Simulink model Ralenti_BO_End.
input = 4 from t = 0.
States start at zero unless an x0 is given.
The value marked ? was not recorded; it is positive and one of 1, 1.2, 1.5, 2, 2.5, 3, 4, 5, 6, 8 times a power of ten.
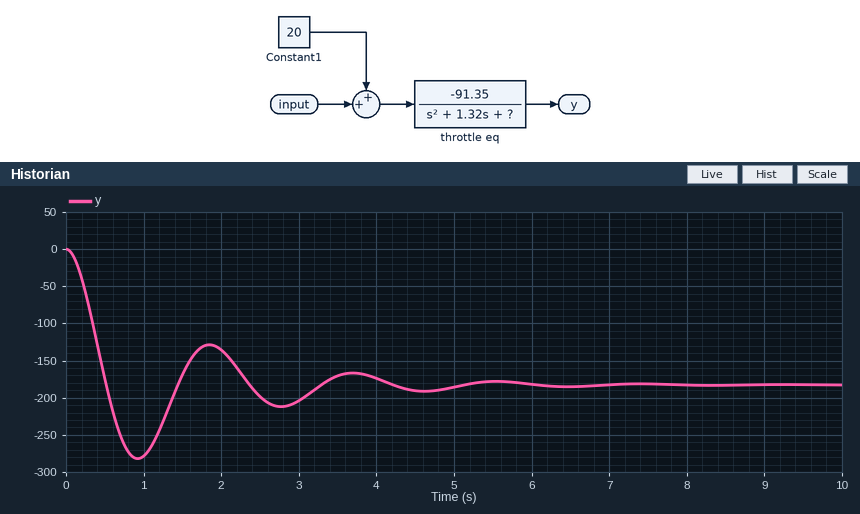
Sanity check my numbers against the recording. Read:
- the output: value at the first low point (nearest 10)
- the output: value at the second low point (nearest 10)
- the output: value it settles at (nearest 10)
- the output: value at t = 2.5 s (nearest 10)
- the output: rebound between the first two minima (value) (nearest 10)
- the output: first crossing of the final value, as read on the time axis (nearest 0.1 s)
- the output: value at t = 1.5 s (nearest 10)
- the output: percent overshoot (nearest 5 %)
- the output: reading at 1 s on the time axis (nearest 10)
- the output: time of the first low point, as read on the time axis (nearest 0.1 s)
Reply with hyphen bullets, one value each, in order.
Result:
- -280
- -210
- -180
- -200
- -130
- 0.5 s
- -170
- 55 %
- -280
- 0.9 s
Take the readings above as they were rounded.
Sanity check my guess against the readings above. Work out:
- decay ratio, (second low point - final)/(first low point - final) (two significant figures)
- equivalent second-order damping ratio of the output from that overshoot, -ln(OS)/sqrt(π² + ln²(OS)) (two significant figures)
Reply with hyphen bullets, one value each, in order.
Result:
- 0.30
- 0.19
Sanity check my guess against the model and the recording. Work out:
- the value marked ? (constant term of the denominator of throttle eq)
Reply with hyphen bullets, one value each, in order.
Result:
- 12
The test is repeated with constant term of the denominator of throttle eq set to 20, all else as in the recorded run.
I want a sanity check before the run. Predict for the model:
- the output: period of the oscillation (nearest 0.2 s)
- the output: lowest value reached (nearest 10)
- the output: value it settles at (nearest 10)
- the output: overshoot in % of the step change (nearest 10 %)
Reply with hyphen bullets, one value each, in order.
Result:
- 1.4 s
- -180
- -110
- 60 %
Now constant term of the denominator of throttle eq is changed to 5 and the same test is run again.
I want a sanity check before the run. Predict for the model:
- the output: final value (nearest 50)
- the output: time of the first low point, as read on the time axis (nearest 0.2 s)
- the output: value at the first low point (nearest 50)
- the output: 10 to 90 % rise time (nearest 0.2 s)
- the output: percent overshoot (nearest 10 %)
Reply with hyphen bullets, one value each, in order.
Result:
- -450
- 1.4 s
- -600
- 0.6 s
- 40 %
